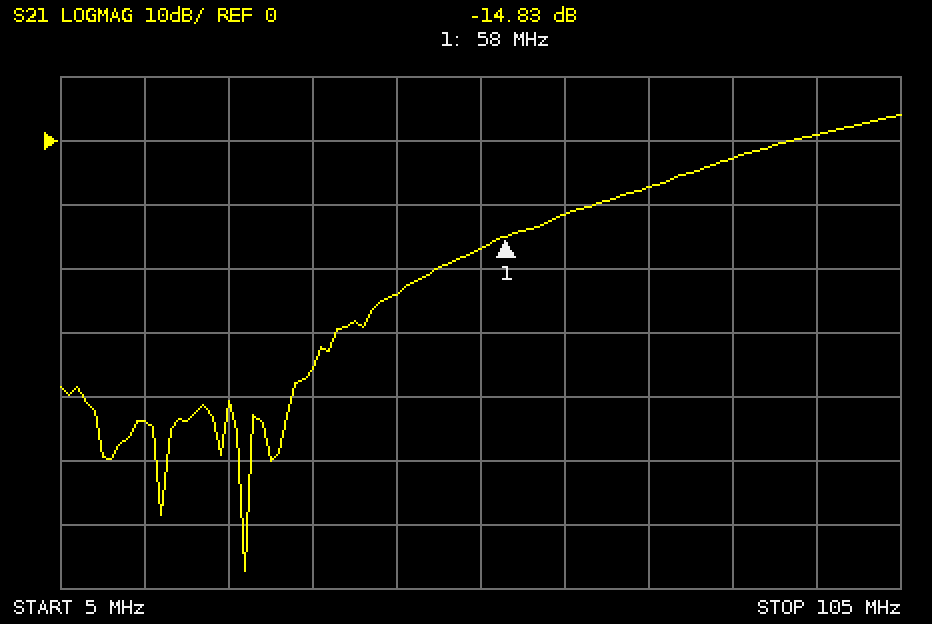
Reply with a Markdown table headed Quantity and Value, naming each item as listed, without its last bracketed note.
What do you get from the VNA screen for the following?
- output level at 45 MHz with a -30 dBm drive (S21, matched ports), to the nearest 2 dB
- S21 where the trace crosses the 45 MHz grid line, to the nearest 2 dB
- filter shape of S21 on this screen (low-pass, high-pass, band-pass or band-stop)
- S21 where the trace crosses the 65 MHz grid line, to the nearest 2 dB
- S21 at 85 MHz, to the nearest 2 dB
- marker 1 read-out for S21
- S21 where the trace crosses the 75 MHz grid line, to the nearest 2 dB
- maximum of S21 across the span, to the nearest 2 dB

| Quantity | Value |
|---|---|
| output level at 45 MHz with a -30 dBm drive (S21, matched ports), to the nearest 2 dB | -54 dBm |
| S21 where the trace crosses the 45 MHz grid line, to the nearest 2 dB | -24 dB |
| filter shape of S21 on this screen | high-pass |
| S21 where the trace crosses the 65 MHz grid line, to the nearest 2 dB | -12 dB |
| S21 at 85 MHz, to the nearest 2 dB | -2 dB |
| marker 1 read-out for S21 | -14.83 dB |
| S21 where the trace crosses the 75 MHz grid line, to the nearest 2 dB | -8 dB |
| maximum of S21 across the span, to the nearest 2 dB | 4 dB |
